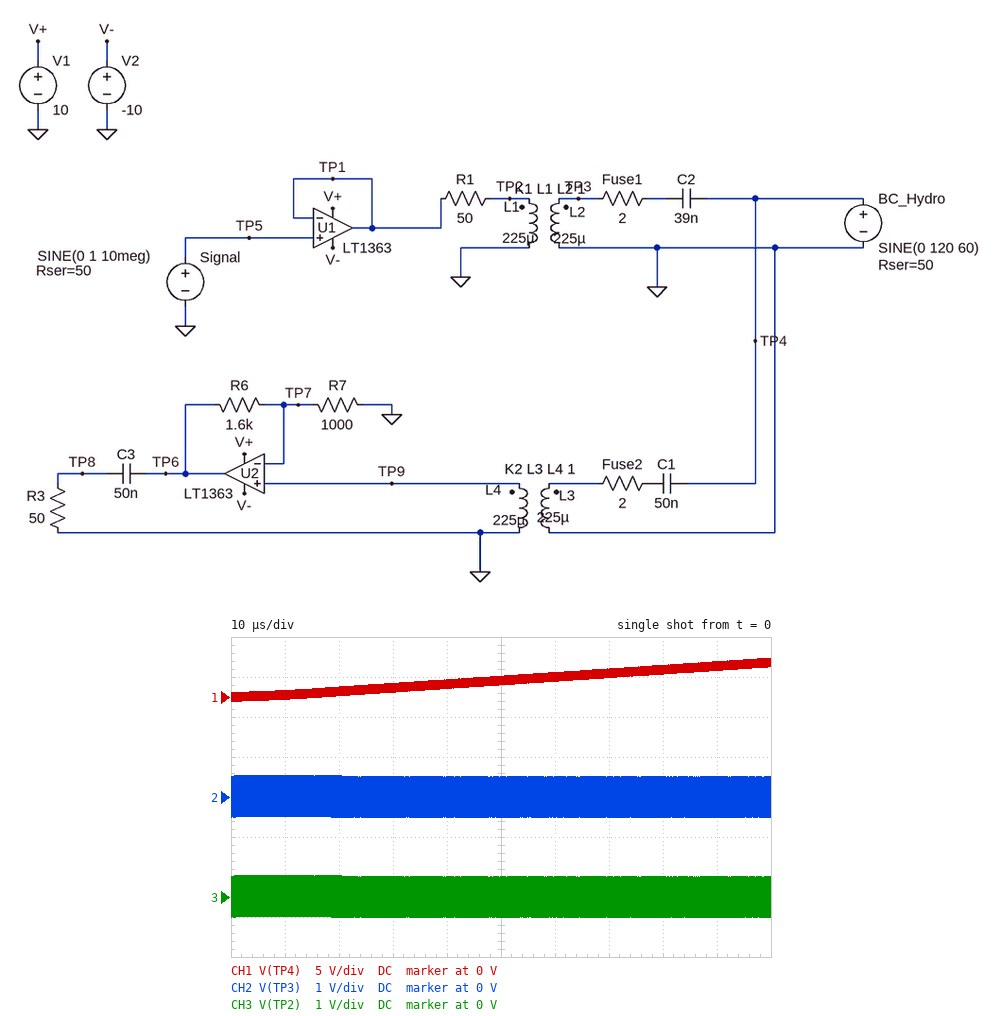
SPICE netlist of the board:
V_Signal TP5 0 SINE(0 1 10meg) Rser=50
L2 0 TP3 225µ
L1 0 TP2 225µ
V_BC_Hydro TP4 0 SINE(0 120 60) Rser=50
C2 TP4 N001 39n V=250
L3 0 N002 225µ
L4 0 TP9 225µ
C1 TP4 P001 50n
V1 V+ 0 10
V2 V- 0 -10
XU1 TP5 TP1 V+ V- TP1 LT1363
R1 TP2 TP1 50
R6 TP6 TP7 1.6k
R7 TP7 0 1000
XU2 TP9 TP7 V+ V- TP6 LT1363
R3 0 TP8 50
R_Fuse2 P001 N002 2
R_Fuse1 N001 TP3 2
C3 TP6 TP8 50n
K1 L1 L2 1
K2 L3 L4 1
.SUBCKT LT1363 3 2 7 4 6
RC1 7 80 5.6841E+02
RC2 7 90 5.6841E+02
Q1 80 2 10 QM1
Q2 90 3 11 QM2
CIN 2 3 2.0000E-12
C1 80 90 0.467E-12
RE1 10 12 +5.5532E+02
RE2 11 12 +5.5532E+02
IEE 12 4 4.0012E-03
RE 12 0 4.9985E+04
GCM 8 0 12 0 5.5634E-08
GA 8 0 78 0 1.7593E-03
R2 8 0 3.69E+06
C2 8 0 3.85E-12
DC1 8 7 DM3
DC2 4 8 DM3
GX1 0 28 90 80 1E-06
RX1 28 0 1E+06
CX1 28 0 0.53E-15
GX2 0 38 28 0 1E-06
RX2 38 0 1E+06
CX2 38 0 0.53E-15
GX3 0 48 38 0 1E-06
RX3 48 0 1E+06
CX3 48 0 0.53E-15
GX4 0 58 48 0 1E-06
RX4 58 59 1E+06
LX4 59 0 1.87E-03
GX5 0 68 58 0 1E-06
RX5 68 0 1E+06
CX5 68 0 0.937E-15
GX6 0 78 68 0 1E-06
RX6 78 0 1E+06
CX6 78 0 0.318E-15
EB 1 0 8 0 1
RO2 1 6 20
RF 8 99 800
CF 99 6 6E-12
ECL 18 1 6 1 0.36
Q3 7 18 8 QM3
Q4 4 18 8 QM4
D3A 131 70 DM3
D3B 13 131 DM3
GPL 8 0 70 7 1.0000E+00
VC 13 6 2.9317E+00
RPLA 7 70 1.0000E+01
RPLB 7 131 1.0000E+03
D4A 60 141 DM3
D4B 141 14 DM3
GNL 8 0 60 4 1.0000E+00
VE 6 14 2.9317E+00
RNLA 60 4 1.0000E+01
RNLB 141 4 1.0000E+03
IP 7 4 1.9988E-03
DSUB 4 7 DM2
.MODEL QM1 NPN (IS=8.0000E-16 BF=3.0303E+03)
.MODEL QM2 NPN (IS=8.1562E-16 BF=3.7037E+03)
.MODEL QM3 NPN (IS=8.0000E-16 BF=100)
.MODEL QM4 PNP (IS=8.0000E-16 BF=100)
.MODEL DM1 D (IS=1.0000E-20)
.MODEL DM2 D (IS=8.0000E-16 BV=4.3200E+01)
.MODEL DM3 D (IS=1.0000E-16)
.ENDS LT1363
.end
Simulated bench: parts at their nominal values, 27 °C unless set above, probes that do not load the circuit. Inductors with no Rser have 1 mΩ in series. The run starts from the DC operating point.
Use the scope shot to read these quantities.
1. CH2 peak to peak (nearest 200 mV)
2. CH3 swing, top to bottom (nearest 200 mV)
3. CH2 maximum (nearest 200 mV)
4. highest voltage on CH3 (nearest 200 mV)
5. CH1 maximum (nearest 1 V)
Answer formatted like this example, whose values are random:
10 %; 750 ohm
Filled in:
1.0 V; 1.0 V; 600 mV; 600 mV; 5 V
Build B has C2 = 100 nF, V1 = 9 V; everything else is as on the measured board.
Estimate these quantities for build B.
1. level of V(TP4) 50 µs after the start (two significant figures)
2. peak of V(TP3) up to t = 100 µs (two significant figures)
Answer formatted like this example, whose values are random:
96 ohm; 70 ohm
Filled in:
1.8 V; 550 mV
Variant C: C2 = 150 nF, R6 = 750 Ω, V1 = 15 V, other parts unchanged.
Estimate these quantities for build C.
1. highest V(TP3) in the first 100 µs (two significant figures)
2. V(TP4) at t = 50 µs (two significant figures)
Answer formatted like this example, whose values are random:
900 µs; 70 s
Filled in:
570 mV; 1.7 V
